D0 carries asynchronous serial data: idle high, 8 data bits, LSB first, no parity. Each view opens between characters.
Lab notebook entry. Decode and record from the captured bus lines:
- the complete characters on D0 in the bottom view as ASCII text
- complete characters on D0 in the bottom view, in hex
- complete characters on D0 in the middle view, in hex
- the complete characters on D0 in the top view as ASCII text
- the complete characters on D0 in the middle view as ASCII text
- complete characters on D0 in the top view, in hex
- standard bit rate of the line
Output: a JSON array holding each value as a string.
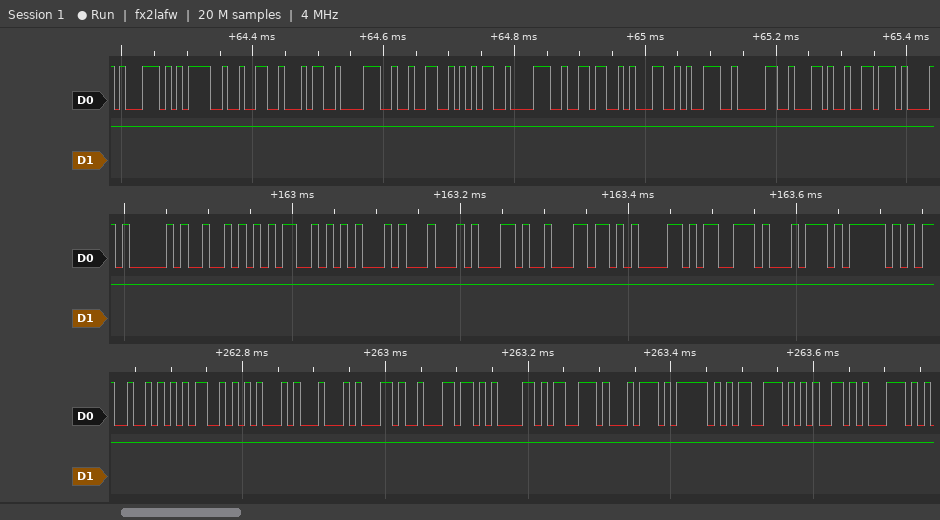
["\"RMED,last_seq\"", "52, 4D, 45, 44, 2C, 6C, 61, 73, 74, 5F, 73, 65, 71", "41, 52, 4D, 45, 44, 2C, 6C, 61, 73, 74, 5F", "\"q=2482586190,v\"", "\"ARMED,last_\"", "71, 3D, 32, 34, 38, 32, 35, 38, 36, 31, 39, 30, 2C, 76", "115200 baud"]
